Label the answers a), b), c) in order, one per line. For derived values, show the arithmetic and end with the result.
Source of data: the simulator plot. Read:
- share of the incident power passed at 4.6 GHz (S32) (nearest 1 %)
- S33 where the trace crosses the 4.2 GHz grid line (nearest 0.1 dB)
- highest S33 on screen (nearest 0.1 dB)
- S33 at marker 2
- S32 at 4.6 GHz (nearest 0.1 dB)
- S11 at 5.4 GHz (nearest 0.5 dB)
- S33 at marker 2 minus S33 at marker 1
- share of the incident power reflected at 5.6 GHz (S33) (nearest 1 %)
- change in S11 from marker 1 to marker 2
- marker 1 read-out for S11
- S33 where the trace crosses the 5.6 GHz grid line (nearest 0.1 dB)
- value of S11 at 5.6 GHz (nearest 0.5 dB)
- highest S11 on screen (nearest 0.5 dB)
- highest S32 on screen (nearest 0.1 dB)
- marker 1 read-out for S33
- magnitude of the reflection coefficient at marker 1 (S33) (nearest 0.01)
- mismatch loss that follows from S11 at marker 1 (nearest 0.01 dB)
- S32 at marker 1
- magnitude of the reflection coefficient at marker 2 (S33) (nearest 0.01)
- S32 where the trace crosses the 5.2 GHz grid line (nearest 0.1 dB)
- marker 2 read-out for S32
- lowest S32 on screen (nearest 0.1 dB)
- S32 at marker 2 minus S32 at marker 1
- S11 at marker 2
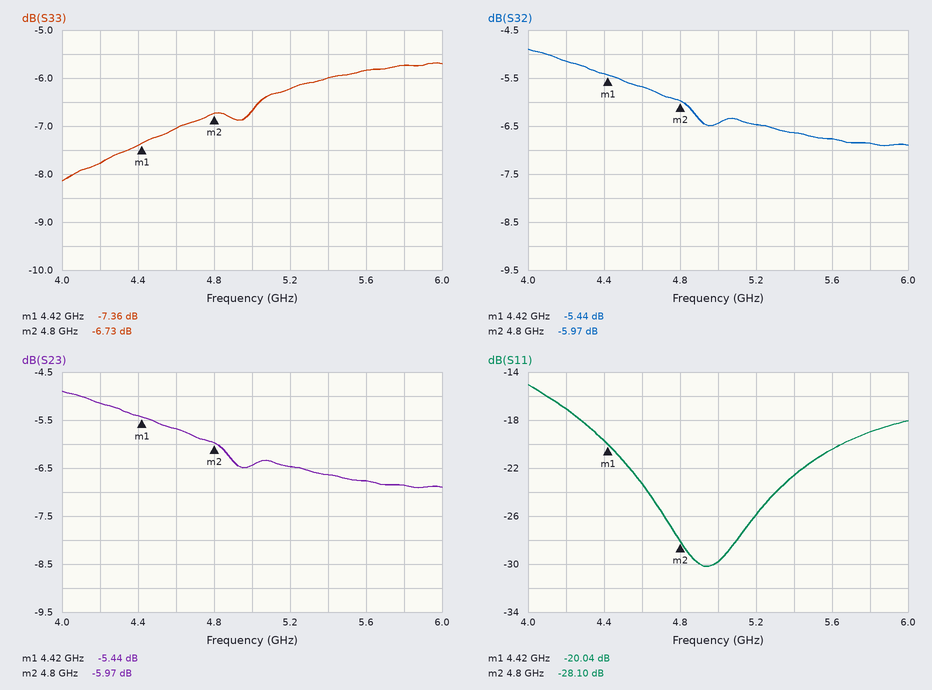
a) 10^(-5.7/10) ≈ 27 %
b) -7.8 dB
c) -5.7 dB
d) -6.73 dB
e) -5.7 dB
f) -22.5 dB
g) -6.73 − (-7.36) = 0.63 dB
h) 10^(-5.8/10) ≈ 26 %
i) -28.1 − (-20.04) = -8.06 dB
j) -20.04 dB
k) -5.8 dB
l) -20.5 dB
m) -15.0 dB
n) -4.9 dB
o) -7.36 dB
p) 10^(-7.36/20) ≈ 0.43
q) −10 log10(1 − 10^(-20.04/10)) ≈ 0.04 dB
r) -5.44 dB
s) 10^(-6.73/20) ≈ 0.46
t) -6.5 dB
u) -5.97 dB
v) -6.9 dB
w) -5.97 − (-5.44) = -0.53 dB
x) -28.10 dB
